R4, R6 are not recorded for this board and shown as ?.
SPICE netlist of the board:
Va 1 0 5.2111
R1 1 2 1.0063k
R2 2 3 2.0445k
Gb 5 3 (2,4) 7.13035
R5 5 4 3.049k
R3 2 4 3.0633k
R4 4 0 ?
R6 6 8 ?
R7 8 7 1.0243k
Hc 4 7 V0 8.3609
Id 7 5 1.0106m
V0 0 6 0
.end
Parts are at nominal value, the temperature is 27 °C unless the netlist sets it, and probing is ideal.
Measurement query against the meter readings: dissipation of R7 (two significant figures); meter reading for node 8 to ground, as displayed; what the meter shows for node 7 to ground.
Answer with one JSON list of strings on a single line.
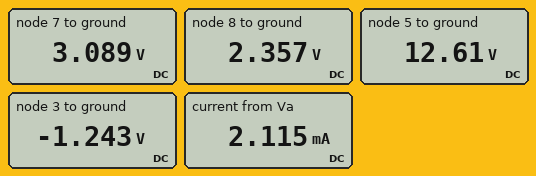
["520 µW", "2.357 V", "3.089 V"]
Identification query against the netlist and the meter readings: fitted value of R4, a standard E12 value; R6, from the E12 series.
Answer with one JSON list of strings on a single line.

["2.2 kΩ", "3.3 kΩ"]
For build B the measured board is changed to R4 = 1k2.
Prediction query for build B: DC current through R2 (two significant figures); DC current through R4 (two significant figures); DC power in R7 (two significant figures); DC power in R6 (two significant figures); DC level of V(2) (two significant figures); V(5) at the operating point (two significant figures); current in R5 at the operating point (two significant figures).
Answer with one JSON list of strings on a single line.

["2.7 mA", "2.1 mA", "350 µW", "1.1 mW", "2.5 V", "14 V", "3.7 mA"]
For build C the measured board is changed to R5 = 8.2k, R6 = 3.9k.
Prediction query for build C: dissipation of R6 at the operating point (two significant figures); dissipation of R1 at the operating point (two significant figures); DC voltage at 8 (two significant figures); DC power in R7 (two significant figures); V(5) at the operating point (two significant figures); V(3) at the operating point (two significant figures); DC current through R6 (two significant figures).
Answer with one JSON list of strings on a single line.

["1.6 mW", "4.3 mW", "2.5 V", "420 µW", "28 V", "-1.1 V", "640 µA"]
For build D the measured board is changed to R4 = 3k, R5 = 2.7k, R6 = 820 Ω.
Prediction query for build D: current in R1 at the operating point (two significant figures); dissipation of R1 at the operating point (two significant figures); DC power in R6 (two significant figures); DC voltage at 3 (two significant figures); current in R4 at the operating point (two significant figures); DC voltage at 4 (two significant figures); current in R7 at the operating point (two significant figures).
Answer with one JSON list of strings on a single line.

["2.4 mA", "5.9 mW", "1.9 mW", "-2.2 V", "920 µA", "2.8 V", "1.5 mA"]
